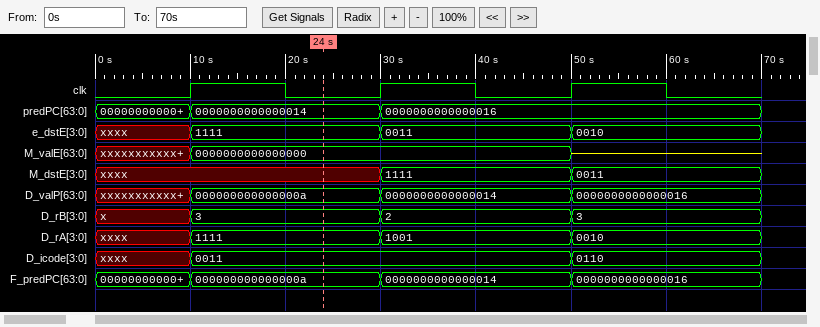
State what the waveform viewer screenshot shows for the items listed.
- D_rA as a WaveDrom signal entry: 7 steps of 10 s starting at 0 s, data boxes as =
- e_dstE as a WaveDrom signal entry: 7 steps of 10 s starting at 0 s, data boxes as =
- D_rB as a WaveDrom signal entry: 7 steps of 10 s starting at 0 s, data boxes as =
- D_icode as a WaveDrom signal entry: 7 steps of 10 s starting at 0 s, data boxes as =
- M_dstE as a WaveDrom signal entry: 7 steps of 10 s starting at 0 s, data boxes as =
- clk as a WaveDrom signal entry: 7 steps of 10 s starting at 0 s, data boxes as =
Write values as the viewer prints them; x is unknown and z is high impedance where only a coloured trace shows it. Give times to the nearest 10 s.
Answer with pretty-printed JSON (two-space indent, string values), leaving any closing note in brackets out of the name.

{
  "D_rA as a WaveDrom signal entry: 7 steps of 10 s starting at 0 s, data boxes as =": "{name: 'D_rA', wave: 'x=.=.=.', data: '1111 1001 0010'}",
  "e_dstE as a WaveDrom signal entry: 7 steps of 10 s starting at 0 s, data boxes as =": "{name: 'e_dstE', wave: 'x=.=.=.', data: '1111 0011 0010'}",
  "D_rB as a WaveDrom signal entry: 7 steps of 10 s starting at 0 s, data boxes as =": "{name: 'D_rB', wave: 'x=.=.=.', data: '3 2 3'}",
  "D_icode as a WaveDrom signal entry: 7 steps of 10 s starting at 0 s, data boxes as =": "{name: 'D_icode', wave: 'x=...=.', data: '0011 0110'}",
  "M_dstE as a WaveDrom signal entry: 7 steps of 10 s starting at 0 s, data boxes as =": "{name: 'M_dstE', wave: 'x..=.=.', data: '1111 0011'}",
  "clk as a WaveDrom signal entry: 7 steps of 10 s starting at 0 s, data boxes as =": "{name: 'clk', wave: '0101010'}"
}
